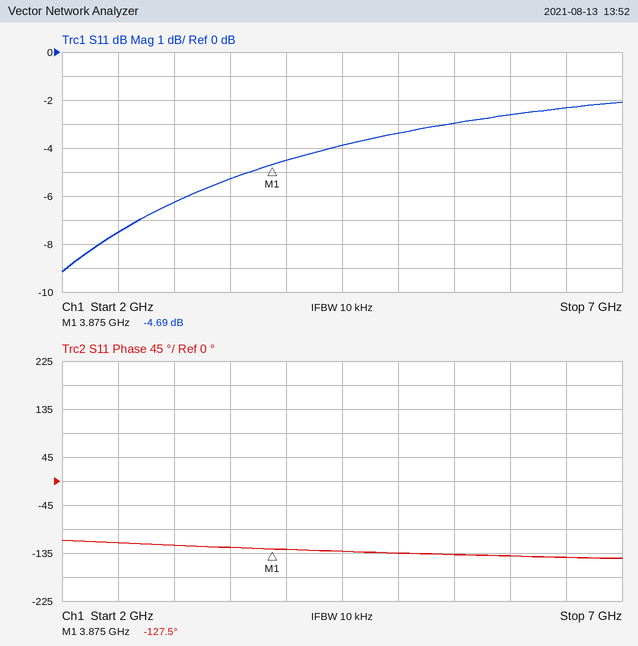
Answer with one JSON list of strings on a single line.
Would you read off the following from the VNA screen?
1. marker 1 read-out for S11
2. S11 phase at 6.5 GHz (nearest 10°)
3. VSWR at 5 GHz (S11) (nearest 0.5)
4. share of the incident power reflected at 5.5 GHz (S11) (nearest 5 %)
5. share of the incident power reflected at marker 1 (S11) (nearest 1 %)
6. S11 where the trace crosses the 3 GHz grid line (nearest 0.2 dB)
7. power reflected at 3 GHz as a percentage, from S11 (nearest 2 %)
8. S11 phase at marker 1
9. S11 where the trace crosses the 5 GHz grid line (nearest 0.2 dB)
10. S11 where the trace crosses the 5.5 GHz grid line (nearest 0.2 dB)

["-4.69 dB", "-140°", "5.0", "50 %", "34 %", "-6.2 dB", "24 %", "-127.5°", "-3.4 dB", "-3.0 dB"]
